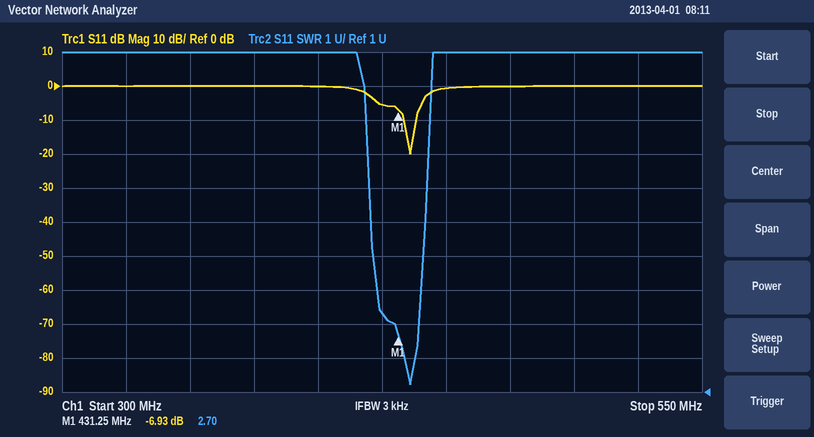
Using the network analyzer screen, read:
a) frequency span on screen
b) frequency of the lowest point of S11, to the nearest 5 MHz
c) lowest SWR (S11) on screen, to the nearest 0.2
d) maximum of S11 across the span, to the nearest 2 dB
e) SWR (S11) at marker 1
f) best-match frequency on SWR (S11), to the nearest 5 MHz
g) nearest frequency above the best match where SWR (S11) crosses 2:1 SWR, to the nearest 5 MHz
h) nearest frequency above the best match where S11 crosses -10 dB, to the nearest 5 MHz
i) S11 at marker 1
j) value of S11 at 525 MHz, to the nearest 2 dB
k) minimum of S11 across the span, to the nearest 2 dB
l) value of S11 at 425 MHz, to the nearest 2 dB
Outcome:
250 MHz
435 MHz
1.2
0 dB
2.70
435 MHz
440 MHz
440 MHz
-6.93 dB
0 dB
-20 dB
-6 dB
